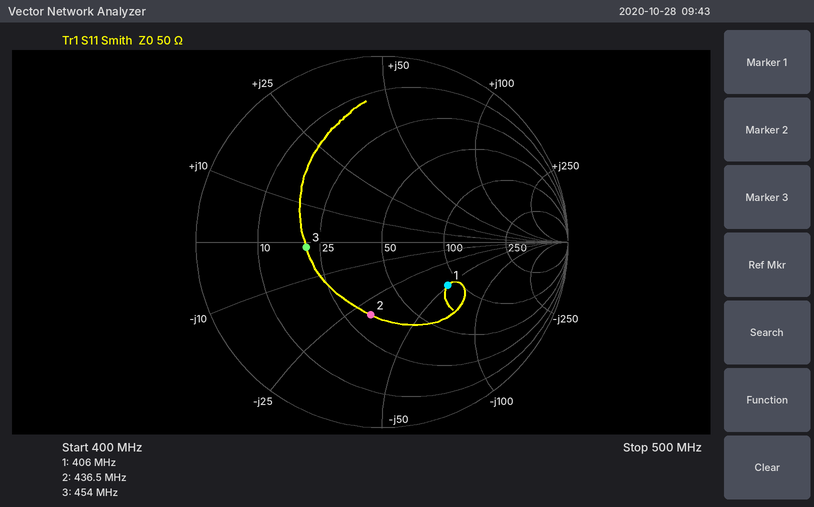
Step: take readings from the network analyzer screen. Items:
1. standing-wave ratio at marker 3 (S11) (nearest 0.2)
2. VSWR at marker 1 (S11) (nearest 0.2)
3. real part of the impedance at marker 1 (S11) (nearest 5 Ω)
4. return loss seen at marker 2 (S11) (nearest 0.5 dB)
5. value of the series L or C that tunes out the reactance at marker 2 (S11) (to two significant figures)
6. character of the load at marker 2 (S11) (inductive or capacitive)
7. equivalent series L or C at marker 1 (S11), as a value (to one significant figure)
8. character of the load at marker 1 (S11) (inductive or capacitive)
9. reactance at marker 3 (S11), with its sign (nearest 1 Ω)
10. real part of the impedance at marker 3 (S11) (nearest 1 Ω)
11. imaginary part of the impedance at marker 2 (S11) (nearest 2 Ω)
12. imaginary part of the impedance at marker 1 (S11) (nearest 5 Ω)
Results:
2.4
2.4
85 Ω
8.0 dB
11 nH
capacitive
8 pF
capacitive
-1 Ω
21 Ω
-30 Ω
-50 Ω
